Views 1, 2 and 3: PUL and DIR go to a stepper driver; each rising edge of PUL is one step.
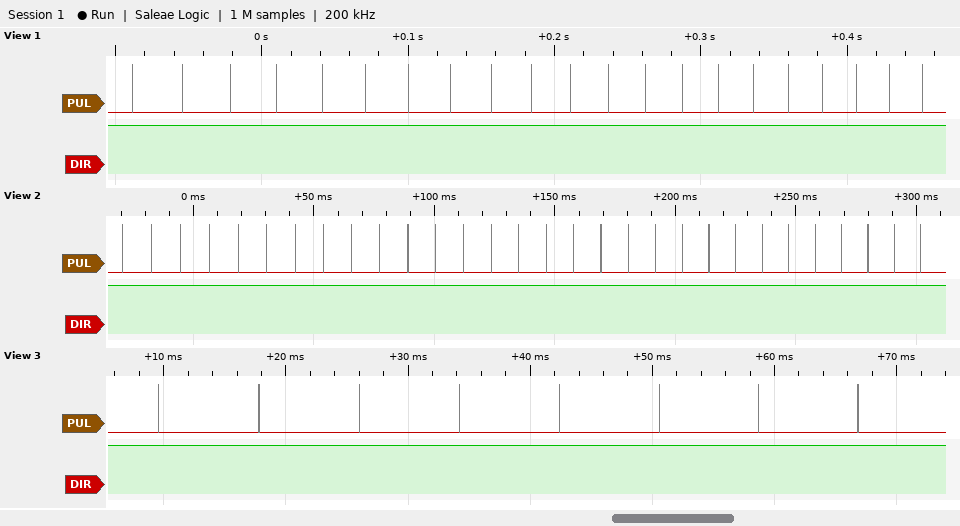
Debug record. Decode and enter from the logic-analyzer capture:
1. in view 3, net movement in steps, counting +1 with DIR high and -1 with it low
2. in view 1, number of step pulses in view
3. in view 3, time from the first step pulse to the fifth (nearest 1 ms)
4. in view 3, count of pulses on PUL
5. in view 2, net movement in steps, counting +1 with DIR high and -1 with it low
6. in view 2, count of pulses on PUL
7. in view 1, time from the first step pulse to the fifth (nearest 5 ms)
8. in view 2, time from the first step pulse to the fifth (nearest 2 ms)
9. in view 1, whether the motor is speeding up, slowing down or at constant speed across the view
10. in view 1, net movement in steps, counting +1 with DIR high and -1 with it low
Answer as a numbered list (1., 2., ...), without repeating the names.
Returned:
1. +8
2. 21
3. 33 ms
4. 8
5. +30
6. 30
7. 130 ms
8. 48 ms
9. speeding up
10. +21
